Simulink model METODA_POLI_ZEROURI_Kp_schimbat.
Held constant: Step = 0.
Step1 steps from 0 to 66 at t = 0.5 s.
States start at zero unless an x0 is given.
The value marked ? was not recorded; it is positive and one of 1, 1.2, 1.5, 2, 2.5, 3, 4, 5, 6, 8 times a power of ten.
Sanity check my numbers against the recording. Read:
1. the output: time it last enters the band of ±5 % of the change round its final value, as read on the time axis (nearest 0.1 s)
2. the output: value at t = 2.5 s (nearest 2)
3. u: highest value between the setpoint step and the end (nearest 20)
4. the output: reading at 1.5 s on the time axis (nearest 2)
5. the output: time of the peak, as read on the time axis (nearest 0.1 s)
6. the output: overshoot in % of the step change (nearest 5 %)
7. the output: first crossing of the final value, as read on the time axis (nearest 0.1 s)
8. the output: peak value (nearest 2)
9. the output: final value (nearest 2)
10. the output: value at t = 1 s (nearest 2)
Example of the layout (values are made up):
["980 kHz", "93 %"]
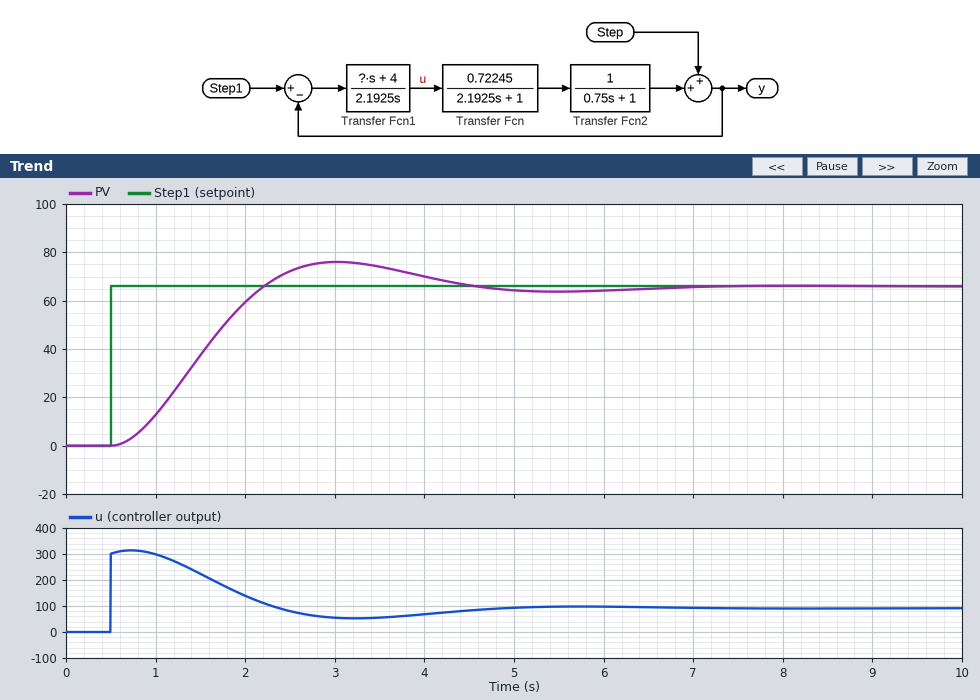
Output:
["4.1 s", "72", "320", "38", "3.0 s", "15 %", "2.2 s", "76", "66", "12"]
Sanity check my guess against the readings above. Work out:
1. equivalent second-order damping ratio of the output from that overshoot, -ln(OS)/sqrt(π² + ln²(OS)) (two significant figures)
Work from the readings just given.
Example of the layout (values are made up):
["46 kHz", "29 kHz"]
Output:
["0.52"]
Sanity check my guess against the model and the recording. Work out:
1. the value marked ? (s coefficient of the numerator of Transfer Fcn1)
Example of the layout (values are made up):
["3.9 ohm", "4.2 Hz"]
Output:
["10"]
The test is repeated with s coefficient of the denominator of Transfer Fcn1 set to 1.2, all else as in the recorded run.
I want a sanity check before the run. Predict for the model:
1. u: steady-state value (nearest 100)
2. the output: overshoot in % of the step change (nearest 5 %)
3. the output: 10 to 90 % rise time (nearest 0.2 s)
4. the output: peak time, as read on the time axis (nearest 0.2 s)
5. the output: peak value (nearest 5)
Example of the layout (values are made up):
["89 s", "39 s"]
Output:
["100", "30 %", "0.8 s", "2.2 s", "85"]
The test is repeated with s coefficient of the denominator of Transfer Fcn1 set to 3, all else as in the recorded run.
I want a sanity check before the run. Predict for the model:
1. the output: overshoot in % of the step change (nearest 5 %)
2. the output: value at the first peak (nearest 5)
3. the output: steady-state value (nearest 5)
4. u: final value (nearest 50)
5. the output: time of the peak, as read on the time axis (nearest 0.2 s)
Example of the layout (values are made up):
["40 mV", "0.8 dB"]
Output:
["10 %", "70", "65", "100", "3.6 s"]
